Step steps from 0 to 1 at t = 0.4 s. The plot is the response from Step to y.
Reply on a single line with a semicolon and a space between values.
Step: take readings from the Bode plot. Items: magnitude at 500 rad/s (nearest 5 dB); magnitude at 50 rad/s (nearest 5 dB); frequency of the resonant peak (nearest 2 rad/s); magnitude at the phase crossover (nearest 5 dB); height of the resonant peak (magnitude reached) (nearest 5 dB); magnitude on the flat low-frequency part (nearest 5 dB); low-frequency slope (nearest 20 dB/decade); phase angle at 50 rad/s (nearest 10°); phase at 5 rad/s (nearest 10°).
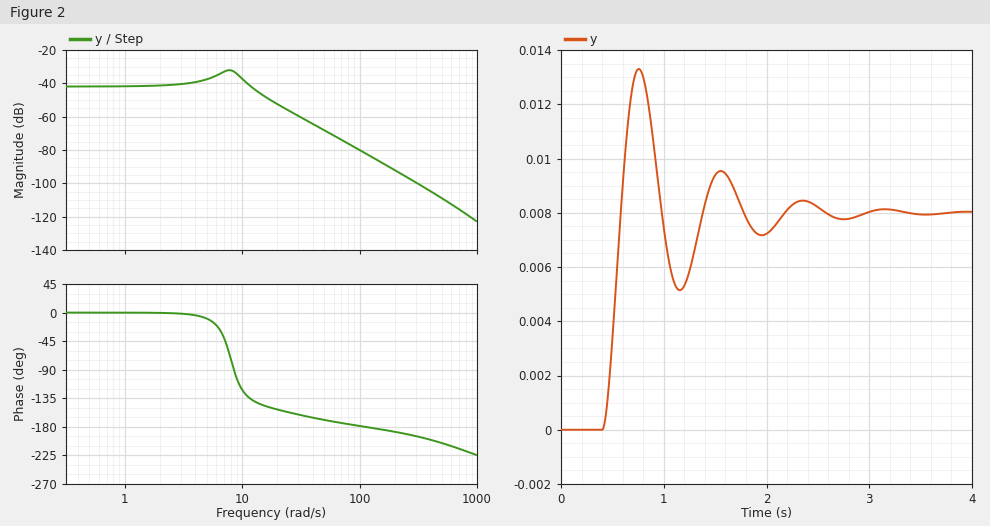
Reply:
-110 dB; -70 dB; 8 rad/s; -80 dB; -30 dB; -40 dB; 0 dB/decade; -170°; -10°
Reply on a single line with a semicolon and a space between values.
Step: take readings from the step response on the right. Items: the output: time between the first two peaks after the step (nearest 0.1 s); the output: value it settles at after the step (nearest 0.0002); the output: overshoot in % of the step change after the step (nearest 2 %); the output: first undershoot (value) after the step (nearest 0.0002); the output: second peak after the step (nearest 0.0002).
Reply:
0.8 s; 0.0080; 66 %; 0.0052; 0.0096
